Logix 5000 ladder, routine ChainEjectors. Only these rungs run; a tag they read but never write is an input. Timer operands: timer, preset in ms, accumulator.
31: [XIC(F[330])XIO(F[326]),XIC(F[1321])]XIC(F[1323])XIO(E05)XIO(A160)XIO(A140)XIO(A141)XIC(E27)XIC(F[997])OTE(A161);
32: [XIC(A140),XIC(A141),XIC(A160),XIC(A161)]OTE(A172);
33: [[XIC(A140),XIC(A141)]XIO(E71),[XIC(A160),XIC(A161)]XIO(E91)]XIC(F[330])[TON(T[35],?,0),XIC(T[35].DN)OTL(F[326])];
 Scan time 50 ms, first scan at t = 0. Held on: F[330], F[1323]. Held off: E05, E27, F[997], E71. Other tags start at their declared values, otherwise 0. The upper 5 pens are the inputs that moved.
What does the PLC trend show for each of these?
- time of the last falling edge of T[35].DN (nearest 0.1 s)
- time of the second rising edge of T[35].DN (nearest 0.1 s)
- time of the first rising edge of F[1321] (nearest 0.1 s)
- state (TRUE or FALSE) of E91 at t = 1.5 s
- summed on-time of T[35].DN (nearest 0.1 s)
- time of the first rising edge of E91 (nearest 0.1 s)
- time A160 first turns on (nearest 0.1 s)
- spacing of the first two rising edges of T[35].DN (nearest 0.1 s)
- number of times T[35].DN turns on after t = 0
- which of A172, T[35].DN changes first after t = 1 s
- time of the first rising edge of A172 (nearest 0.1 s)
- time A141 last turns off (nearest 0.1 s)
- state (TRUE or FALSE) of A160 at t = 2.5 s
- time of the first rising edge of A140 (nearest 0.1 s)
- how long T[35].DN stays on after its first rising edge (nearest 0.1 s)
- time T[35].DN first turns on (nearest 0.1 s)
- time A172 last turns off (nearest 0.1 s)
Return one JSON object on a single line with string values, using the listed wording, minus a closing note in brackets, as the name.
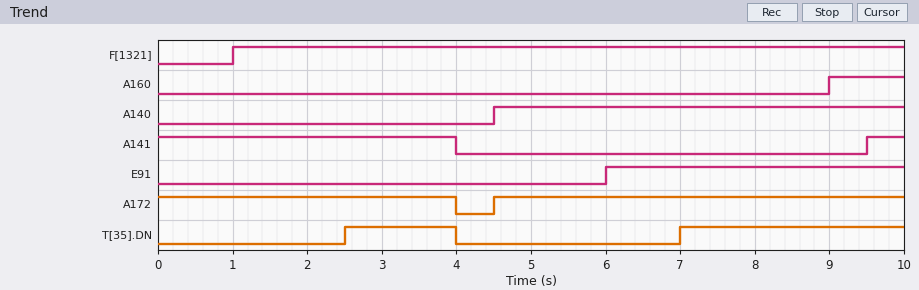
{"time of the last falling edge of T[35].DN": "4.0 s", "time of the second rising edge of T[35].DN": "7.0 s", "time of the first rising edge of F[1321]": "1.0 s", "state (TRUE or FALSE) of E91 at t = 1.5 s": "FALSE", "summed on-time of T[35].DN": "4.5 s", "time of the first rising edge of E91": "6.0 s", "time A160 first turns on": "9.0 s", "spacing of the first two rising edges of T[35].DN": "4.5 s", "number of times T[35].DN turns on after t = 0": "2", "which of A172, T[35].DN changes first after t = 1 s": "T[35].DN", "time of the first rising edge of A172": "4.5 s", "time A141 last turns off": "4.0 s", "state (TRUE or FALSE) of A160 at t = 2.5 s": "FALSE", "time of the first rising edge of A140": "4.5 s", "how long T[35].DN stays on after its first rising edge": "1.5 s", "time T[35].DN first turns on": "2.5 s", "time A172 last turns off": "4.0 s"}
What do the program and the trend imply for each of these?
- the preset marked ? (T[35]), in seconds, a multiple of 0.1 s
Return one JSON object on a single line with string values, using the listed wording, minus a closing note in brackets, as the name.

{"the preset marked ? (T[35]), in seconds, a multiple of 0.1 s": "2.5 s"}
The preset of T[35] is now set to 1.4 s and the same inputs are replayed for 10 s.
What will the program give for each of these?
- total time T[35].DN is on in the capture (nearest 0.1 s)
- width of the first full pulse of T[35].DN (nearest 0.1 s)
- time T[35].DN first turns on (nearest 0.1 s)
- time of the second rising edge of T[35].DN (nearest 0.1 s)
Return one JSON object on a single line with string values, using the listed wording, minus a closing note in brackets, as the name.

{"total time T[35].DN is on in the capture": "6.7 s", "width of the first full pulse of T[35].DN": "2.6 s", "time T[35].DN first turns on": "1.4 s", "time of the second rising edge of T[35].DN": "5.9 s"}
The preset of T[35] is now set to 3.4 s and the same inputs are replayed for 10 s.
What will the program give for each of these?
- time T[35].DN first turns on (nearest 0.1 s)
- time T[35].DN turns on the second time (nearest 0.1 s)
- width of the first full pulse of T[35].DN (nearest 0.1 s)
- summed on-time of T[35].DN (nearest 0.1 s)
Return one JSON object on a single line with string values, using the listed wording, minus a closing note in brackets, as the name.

{"time T[35].DN first turns on": "3.4 s", "time T[35].DN turns on the second time": "7.9 s", "width of the first full pulse of T[35].DN": "0.6 s", "summed on-time of T[35].DN": "2.7 s"}
